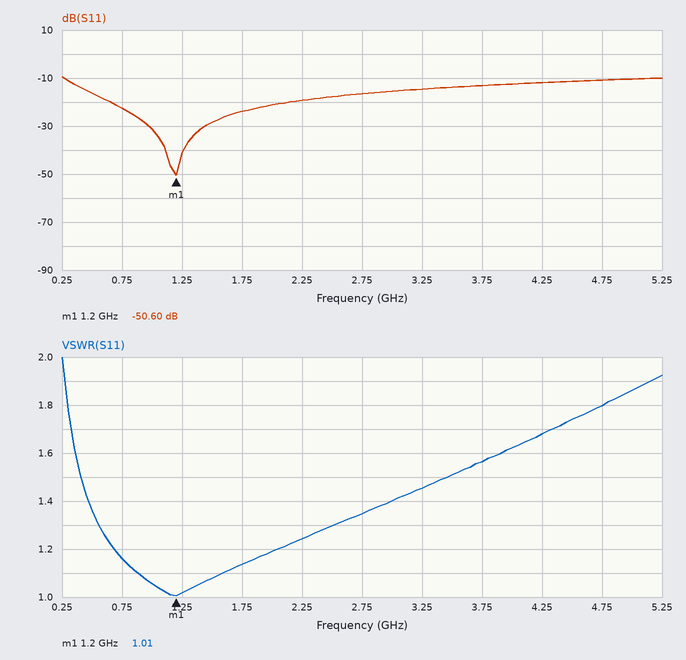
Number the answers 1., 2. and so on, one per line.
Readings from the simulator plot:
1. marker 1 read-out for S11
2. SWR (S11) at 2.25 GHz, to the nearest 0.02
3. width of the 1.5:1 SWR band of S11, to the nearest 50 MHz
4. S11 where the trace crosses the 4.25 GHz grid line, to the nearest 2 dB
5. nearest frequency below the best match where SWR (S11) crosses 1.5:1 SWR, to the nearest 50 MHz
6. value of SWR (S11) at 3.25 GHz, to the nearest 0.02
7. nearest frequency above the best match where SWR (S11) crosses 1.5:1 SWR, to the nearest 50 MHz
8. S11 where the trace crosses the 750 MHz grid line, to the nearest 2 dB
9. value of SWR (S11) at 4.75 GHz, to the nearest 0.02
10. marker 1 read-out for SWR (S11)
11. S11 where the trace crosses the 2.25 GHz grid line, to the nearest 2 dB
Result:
1. -50.60 dB
2. 1.24
3. 3.05 GHz
4. -12 dB
5. 400 MHz
6. 1.46
7. 3.45 GHz
8. -22 dB
9. 1.80
10. 1.01
11. -20 dB
